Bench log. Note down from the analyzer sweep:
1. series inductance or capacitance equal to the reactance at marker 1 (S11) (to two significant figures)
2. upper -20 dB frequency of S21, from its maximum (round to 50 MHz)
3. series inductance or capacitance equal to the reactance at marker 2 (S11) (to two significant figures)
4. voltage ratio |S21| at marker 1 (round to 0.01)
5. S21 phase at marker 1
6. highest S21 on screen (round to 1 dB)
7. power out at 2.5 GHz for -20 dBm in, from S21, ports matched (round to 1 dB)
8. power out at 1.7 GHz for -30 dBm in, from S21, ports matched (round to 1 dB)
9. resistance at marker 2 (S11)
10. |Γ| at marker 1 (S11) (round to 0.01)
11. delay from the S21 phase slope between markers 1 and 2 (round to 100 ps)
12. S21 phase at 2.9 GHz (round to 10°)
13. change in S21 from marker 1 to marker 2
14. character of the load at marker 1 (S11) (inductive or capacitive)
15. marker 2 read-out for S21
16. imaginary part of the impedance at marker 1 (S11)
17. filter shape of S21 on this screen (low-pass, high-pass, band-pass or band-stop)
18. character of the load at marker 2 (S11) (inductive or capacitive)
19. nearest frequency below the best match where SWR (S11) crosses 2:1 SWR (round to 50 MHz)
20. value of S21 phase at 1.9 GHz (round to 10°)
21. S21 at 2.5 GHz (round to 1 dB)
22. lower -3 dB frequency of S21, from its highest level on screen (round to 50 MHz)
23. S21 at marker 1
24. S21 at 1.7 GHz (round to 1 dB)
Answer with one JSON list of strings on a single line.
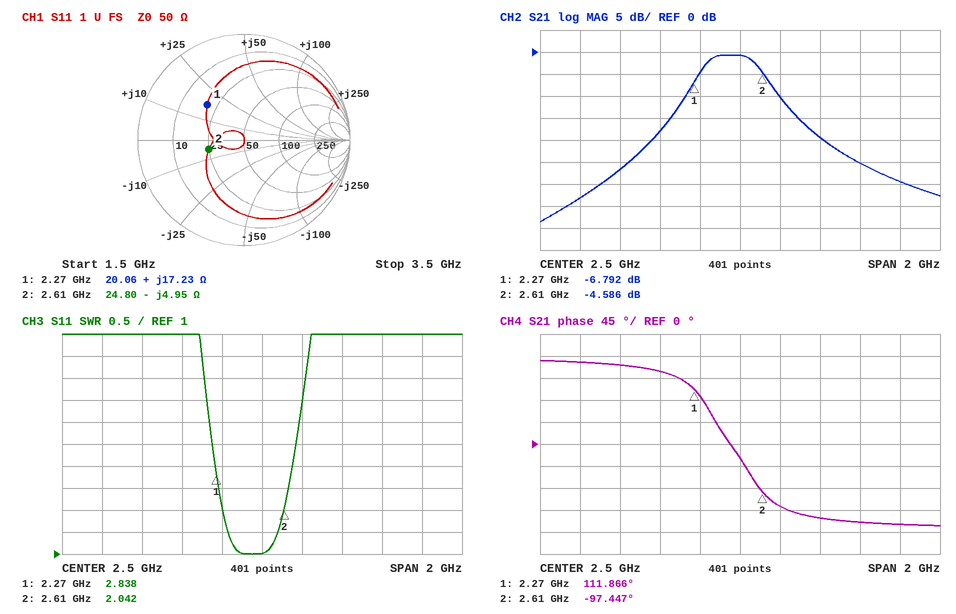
["1.2 nH", "2.95 GHz", "12 pF", "0.46", "111.866°", "-1 dB", "-21 dBm", "-63 dBm", "24.80 Ω", "0.48", "1.7 ns", "-150°", "2.206 dB", "inductive", "-4.586 dB", "+17.23 Ω", "band-pass", "capacitive", "2.30 GHz", "160°", "-1 dB", "2.30 GHz", "-6.792 dB", "-33 dB"]
